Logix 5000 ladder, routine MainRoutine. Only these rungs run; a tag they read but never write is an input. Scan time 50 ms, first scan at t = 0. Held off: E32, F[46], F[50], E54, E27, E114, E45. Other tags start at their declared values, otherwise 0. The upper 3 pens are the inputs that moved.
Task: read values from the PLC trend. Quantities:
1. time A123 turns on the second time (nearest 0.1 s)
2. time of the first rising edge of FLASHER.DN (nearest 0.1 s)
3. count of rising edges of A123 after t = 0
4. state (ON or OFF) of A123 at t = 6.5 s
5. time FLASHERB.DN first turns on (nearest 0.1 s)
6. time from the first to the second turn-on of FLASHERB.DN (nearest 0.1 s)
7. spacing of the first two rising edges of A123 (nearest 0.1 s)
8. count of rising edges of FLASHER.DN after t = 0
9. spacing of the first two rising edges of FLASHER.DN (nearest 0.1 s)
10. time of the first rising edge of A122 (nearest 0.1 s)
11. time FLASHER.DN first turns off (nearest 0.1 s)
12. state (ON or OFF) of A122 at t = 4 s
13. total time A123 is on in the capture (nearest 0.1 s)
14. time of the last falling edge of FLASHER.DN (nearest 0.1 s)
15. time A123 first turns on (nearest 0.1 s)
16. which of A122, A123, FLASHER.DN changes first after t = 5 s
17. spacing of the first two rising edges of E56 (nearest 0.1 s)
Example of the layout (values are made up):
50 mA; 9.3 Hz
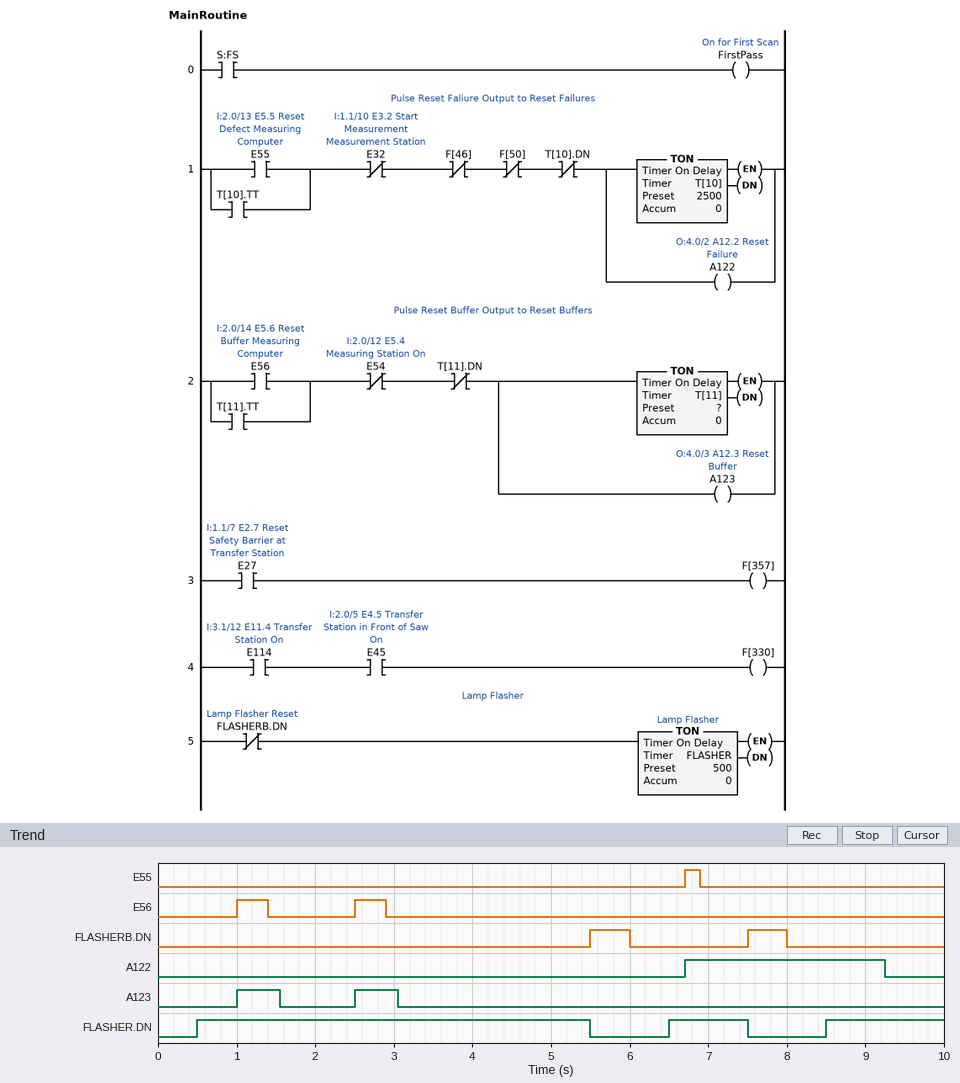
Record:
2.5 s; 0.5 s; 2; OFF; 5.5 s; 2.0 s; 1.5 s; 3; 6.0 s; 6.7 s; 5.5 s; OFF; 1.1 s; 7.5 s; 1.0 s; FLASHER.DN; 1.5 s
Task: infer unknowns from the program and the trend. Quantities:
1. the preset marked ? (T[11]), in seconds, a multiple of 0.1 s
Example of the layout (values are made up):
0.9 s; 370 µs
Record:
0.5 s
